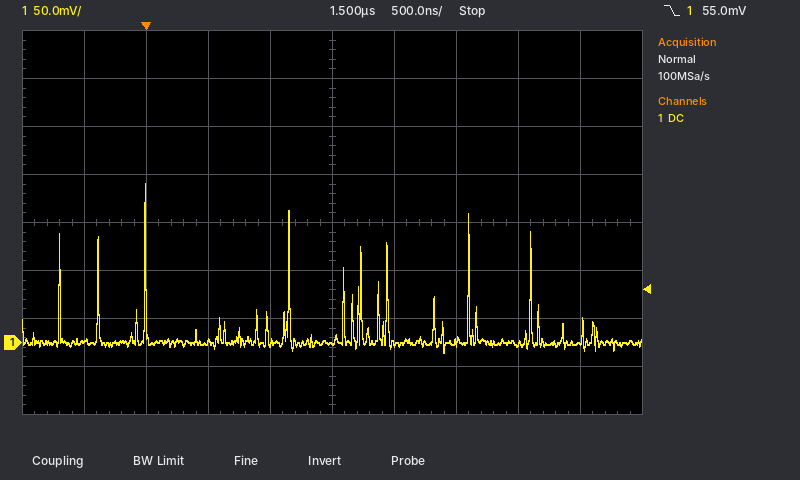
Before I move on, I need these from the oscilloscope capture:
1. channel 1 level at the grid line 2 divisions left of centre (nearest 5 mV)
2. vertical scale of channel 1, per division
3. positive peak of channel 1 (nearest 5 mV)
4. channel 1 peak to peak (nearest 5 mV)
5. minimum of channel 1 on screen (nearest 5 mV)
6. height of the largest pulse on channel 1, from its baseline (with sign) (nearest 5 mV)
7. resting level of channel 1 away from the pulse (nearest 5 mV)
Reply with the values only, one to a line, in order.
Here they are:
0 mV
50 mV
165 mV
175 mV
-10 mV
+165 mV
0 mV
